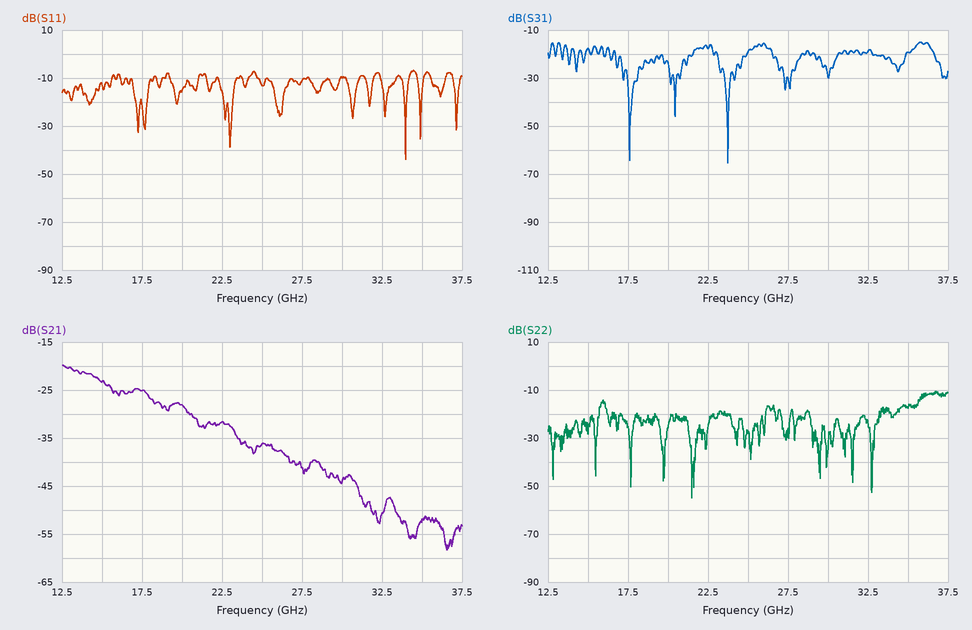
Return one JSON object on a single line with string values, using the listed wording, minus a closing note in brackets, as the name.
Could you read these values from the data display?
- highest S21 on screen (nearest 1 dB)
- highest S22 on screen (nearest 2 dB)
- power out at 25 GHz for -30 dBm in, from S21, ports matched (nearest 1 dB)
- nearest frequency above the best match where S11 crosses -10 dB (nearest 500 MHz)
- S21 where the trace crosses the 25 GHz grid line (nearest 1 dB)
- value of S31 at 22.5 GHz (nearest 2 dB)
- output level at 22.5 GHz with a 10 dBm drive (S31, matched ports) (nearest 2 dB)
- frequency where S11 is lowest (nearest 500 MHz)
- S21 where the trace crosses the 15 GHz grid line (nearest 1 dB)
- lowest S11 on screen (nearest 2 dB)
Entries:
{"highest S21 on screen": "-20 dB", "highest S22 on screen": "-10 dB", "power out at 25 GHz for -30 dBm in, from S21, ports matched": "-66 dBm", "nearest frequency above the best match where S11 crosses -10 dB": "34.0 GHz", "S21 where the trace crosses the 25 GHz grid line": "-36 dB", "value of S31 at 22.5 GHz": "-18 dB", "output level at 22.5 GHz with a 10 dBm drive (S31, matched ports)": "-8 dBm", "frequency where S11 is lowest": "34.0 GHz", "S21 where the trace crosses the 15 GHz grid line": "-23 dB", "lowest S11 on screen": "-44 dB"}
